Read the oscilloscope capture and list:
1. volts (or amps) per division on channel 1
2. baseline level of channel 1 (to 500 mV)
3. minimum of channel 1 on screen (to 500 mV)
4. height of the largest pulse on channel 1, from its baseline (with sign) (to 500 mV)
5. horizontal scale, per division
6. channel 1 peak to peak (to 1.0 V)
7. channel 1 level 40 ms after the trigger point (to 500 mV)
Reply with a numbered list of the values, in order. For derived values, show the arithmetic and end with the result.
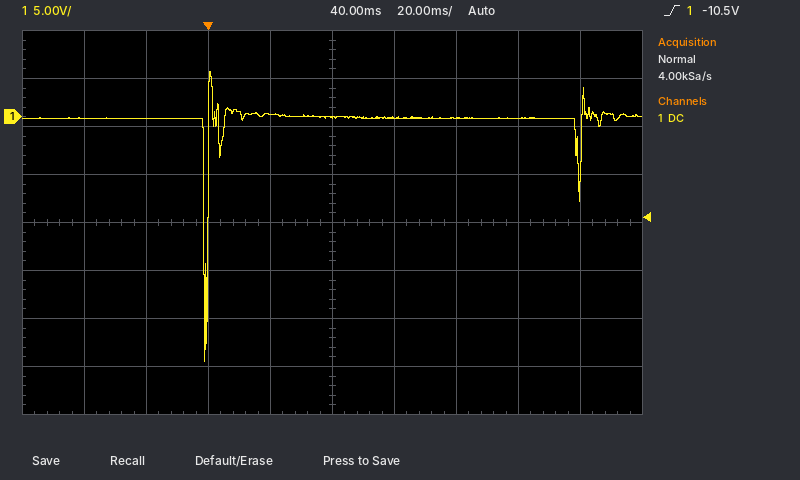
1. 5 V
2. 0.0 V
3. -25.5 V
4. -25.5 V − (0.0 V) = -25.5 V
5. 20 ms
6. 30.0 V
7. 0.0 V
